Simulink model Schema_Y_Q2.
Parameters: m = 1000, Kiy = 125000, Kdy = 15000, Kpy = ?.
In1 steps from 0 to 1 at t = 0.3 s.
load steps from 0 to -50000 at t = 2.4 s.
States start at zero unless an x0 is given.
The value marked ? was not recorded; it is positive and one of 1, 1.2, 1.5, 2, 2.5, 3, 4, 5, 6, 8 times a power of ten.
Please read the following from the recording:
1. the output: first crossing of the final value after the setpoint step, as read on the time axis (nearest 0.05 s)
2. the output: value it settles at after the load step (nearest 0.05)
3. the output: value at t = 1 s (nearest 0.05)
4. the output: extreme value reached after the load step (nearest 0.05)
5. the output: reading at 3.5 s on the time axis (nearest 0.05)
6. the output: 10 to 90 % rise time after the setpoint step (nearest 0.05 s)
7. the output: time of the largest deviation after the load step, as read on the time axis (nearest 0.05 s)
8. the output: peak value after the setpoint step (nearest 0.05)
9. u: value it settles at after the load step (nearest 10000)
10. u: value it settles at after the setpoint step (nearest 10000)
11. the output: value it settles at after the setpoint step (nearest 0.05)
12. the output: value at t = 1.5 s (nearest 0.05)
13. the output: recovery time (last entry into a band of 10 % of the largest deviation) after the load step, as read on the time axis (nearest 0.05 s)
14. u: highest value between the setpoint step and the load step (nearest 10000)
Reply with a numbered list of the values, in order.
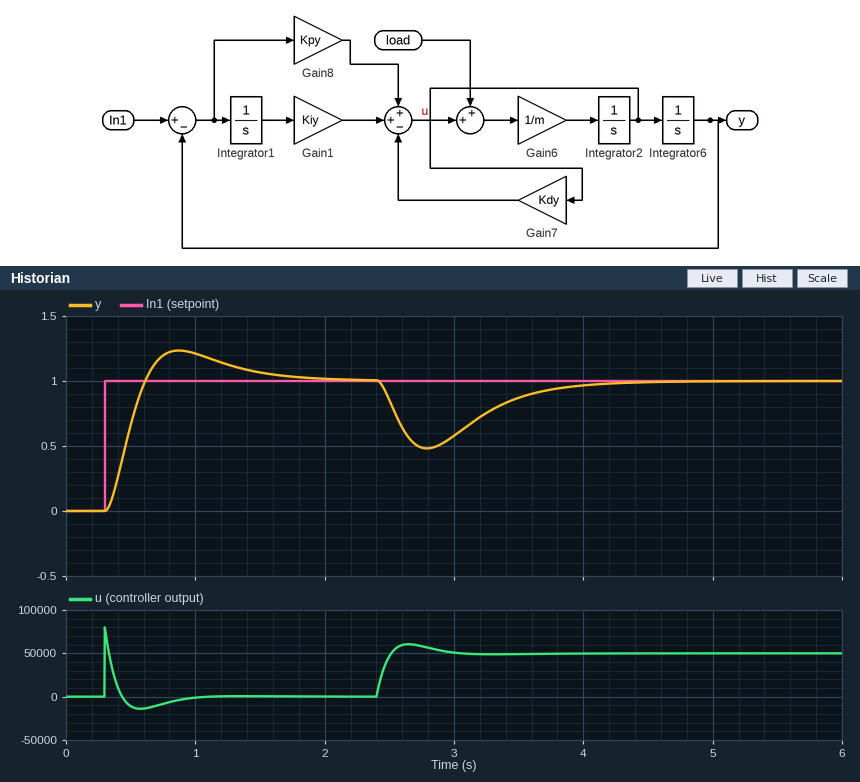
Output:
1. 0.60 s
2. 1.00
3. 1.20
4. 0.50
5. 0.85
6. 0.20 s
7. 2.80 s
8. 1.25
9. 50000
10. 0
11. 1.00
12. 1.05
13. 3.85 s
14. 80000
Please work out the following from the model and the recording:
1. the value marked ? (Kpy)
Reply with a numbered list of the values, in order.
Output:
1. 80000
